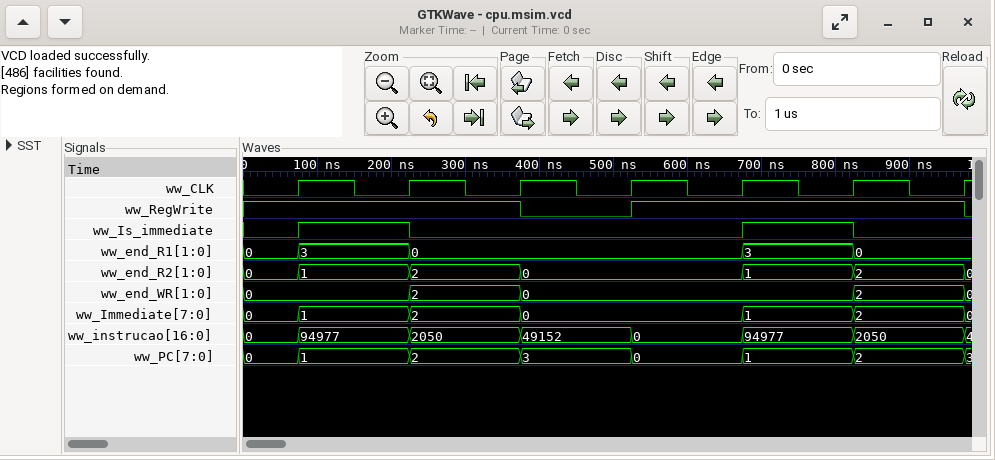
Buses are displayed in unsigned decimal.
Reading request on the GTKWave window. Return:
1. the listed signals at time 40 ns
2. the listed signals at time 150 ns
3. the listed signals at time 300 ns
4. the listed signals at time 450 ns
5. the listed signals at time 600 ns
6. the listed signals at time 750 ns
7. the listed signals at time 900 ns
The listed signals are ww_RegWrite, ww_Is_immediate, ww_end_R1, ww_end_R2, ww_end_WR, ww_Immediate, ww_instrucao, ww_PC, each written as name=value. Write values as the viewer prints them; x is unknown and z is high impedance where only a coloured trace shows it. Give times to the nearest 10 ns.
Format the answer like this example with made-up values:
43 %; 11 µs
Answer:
ww_RegWrite=1, ww_Is_immediate=0, ww_end_R1=0, ww_end_R2=0, ww_end_WR=0, ww_Immediate=0, ww_instrucao=0, ww_PC=0; ww_RegWrite=1, ww_Is_immediate=1, ww_end_R1=3, ww_end_R2=1, ww_end_WR=0, ww_Immediate=1, ww_instrucao=94977, ww_PC=1; ww_RegWrite=1, ww_Is_immediate=0, ww_end_R1=0, ww_end_R2=2, ww_end_WR=2, ww_Immediate=2, ww_instrucao=2050, ww_PC=2; ww_RegWrite=0, ww_Is_immediate=0, ww_end_R1=0, ww_end_R2=0, ww_end_WR=0, ww_Immediate=0, ww_instrucao=49152, ww_PC=3; ww_RegWrite=1, ww_Is_immediate=0, ww_end_R1=0, ww_end_R2=0, ww_end_WR=0, ww_Immediate=0, ww_instrucao=0, ww_PC=0; ww_RegWrite=1, ww_Is_immediate=1, ww_end_R1=3, ww_end_R2=1, ww_end_WR=0, ww_Immediate=1, ww_instrucao=94977, ww_PC=1; ww_RegWrite=1, ww_Is_immediate=0, ww_end_R1=0, ww_end_R2=2, ww_end_WR=2, ww_Immediate=2, ww_instrucao=2050, ww_PC=2
